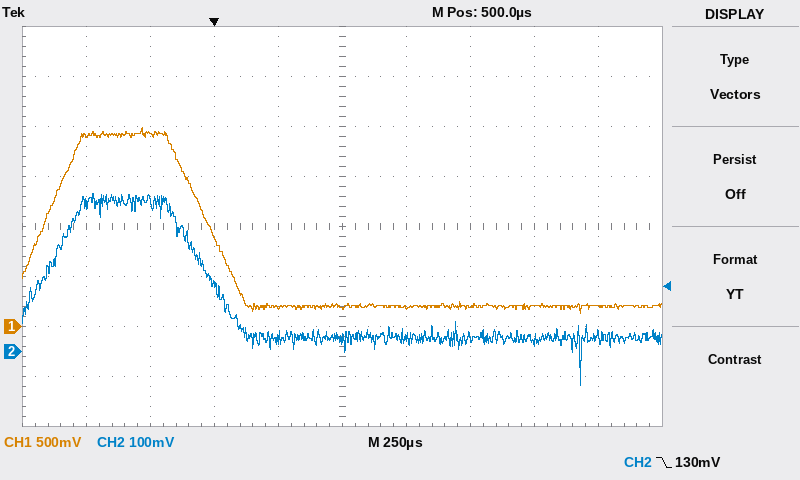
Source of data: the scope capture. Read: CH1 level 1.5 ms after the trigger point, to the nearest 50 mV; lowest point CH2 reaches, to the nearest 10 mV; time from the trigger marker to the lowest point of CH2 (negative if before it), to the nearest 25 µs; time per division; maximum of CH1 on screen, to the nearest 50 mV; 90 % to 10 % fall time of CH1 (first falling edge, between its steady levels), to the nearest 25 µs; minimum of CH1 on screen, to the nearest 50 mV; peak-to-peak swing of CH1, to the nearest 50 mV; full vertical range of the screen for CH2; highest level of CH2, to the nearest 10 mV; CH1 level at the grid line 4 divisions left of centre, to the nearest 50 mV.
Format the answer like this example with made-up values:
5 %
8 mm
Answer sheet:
200 mV
-70 mV
+1.425 ms
250 µs
2.00 V
250 µs
150 mV
1.85 V
800 mV
320 mV
1.90 V
